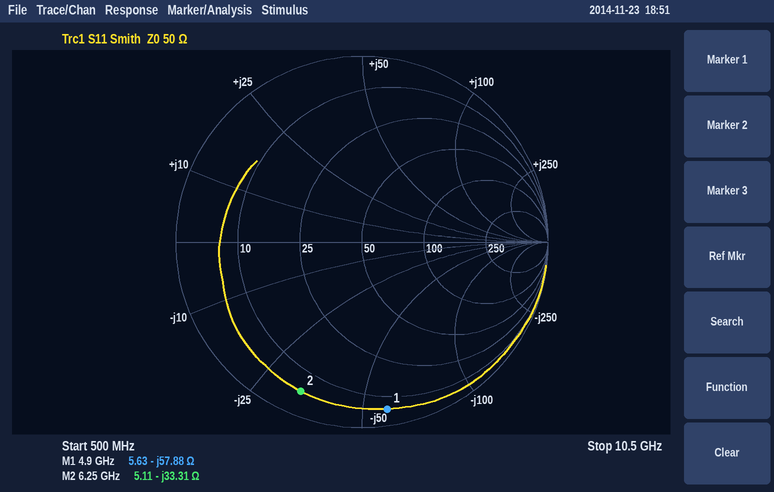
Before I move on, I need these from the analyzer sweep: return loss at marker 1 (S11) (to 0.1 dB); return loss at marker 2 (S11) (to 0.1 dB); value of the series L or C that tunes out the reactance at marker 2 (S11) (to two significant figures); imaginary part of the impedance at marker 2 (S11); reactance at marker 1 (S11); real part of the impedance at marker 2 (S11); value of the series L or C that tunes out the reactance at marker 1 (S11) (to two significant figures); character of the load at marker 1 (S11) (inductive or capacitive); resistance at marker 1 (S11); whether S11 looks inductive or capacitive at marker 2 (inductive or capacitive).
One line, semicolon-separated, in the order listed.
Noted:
0.8 dB; 1.2 dB; 850 pH; -33.31 Ω; -57.88 Ω; 5.11 Ω; 1.9 nH; capacitive; 5.63 Ω; capacitive
